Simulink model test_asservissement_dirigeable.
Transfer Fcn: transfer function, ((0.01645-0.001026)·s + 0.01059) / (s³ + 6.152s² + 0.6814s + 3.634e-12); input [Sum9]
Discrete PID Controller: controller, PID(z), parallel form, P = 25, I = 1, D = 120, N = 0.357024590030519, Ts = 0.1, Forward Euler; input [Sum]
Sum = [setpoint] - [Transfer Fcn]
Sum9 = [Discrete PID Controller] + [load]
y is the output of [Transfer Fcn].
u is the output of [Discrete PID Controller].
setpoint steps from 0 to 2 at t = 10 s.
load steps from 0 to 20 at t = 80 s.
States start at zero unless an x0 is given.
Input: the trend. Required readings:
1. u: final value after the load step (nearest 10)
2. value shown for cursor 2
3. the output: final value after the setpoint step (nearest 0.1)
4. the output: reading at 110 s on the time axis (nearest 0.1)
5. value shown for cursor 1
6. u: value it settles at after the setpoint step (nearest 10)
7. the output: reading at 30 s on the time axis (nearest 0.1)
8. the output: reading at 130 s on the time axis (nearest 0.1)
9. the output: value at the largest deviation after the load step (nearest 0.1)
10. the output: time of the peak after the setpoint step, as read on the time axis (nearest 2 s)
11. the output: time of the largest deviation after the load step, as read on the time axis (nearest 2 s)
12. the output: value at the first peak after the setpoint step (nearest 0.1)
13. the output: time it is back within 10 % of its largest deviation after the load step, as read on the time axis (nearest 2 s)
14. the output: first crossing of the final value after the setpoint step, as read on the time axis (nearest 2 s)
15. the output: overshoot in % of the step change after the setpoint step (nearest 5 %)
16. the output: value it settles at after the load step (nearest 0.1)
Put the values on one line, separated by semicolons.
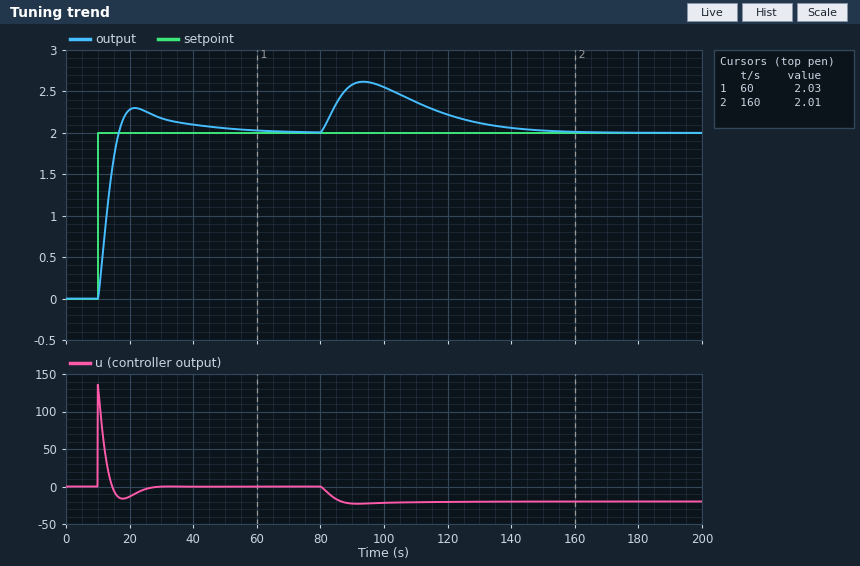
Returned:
-20; 2.01; 2.0; 2.4; 2.03; 0; 2.2; 2.1; 2.6; 22 s; 94 s; 2.3; 140 s; 16 s; 15 %; 2.0
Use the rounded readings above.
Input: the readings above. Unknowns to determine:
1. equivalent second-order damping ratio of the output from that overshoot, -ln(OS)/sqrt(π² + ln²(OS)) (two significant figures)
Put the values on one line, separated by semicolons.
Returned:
0.52
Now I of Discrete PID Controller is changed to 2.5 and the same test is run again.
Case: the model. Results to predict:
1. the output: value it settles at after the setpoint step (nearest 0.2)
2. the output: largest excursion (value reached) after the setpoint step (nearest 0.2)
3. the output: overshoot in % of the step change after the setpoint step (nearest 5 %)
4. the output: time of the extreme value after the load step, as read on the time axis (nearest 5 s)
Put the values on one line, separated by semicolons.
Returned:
2.0; 2.6; 25 %; 90 s
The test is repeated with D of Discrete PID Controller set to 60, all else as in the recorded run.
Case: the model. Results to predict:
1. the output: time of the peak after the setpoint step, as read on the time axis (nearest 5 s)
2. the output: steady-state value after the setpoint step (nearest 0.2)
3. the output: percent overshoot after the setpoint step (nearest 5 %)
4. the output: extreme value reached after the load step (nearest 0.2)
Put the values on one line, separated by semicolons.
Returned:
25 s; 2.0; 25 %; 2.8
